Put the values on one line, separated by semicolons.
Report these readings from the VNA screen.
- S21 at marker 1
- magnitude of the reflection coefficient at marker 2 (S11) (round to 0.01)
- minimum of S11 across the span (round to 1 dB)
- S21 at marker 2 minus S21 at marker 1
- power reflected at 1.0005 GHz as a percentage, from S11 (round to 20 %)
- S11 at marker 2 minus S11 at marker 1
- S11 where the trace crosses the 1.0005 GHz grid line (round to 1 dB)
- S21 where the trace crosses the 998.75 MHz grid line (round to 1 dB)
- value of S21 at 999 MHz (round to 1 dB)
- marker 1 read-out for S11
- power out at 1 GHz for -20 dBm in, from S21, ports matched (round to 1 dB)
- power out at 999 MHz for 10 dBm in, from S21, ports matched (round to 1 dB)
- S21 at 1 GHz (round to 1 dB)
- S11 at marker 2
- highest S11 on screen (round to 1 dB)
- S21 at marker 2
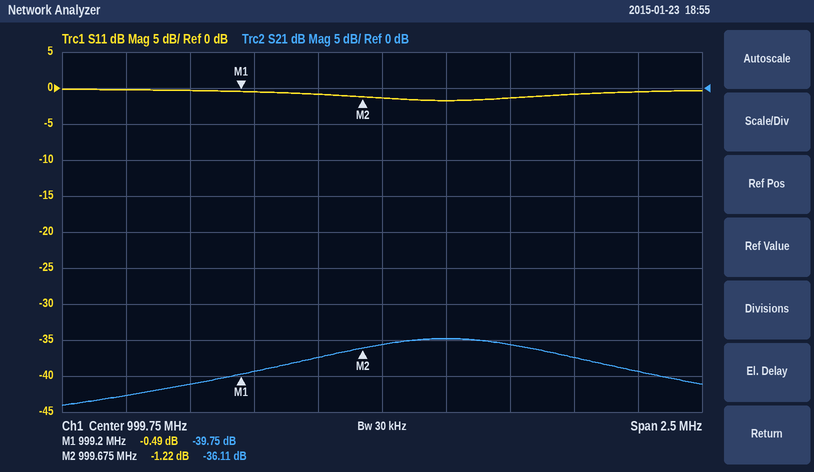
-39.75 dB; 0.87; -2 dB; 3.64 dB; 80 %; -0.73 dB; -1 dB; -43 dB; -41 dB; -0.49 dB; -55 dBm; -31 dBm; -35 dB; -1.22 dB; 0 dB; -36.11 dB
